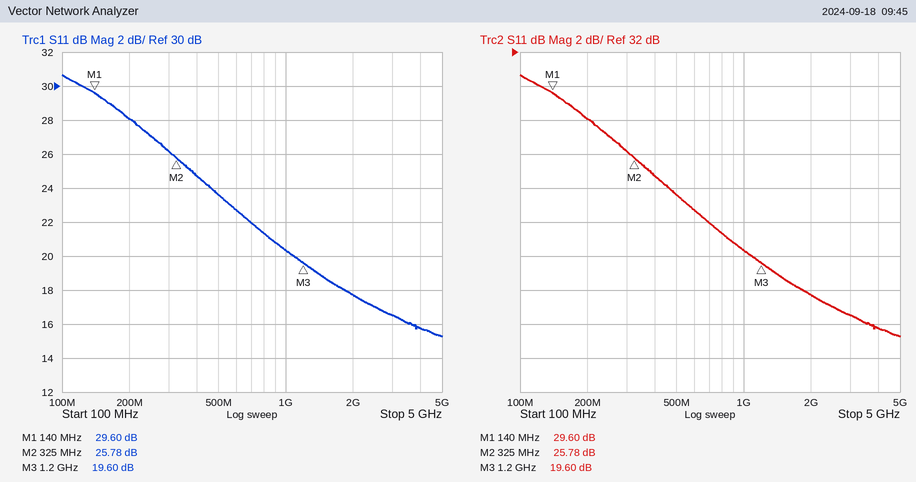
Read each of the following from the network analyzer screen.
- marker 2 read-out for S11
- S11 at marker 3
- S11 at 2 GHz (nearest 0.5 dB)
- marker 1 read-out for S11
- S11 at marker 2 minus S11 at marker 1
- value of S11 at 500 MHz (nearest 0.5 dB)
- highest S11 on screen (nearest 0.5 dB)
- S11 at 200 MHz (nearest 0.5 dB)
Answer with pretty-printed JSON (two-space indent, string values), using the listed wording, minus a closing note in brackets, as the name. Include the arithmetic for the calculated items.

{
  "marker 2 read-out for S11": "25.78 dB",
  "S11 at marker 3": "19.60 dB",
  "S11 at 2 GHz": "17.5 dB",
  "marker 1 read-out for S11": "29.60 dB",
  "S11 at marker 2 minus S11 at marker 1": "25.78 − (29.6) = -3.82 dB",
  "value of S11 at 500 MHz": "23.5 dB",
  "highest S11 on screen": "30.5 dB",
  "S11 at 200 MHz": "28.0 dB"
}
